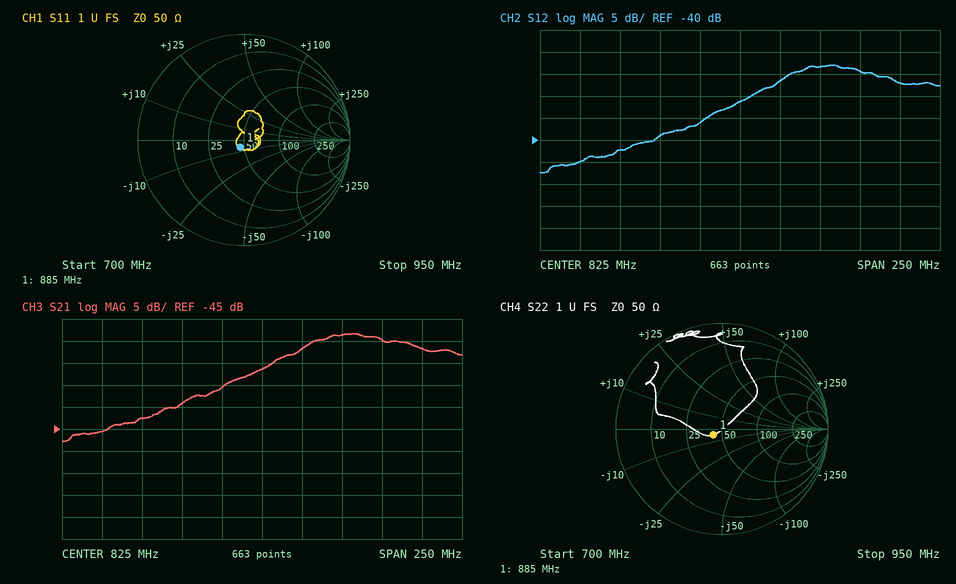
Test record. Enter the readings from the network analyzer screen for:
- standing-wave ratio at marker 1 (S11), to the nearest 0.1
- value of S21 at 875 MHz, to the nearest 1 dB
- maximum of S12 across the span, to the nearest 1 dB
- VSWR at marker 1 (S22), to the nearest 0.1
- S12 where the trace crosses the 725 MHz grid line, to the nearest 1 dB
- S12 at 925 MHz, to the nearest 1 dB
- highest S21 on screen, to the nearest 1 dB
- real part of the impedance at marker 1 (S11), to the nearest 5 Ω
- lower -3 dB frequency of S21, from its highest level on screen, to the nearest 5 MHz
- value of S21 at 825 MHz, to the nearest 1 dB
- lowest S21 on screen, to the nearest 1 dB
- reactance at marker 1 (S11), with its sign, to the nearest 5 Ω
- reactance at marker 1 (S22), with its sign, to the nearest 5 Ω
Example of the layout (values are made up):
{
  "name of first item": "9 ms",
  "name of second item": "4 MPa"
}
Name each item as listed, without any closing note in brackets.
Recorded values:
{
  "standing-wave ratio at marker 1 (S11), to the nearest 0.1": "1.2",
  "value of S21 at 875 MHz, to the nearest 1 dB": "-24 dB",
  "maximum of S12 across the span, to the nearest 1 dB": "-23 dB",
  "VSWR at marker 1 (S22), to the nearest 0.1": "1.2",
  "S12 where the trace crosses the 725 MHz grid line, to the nearest 1 dB": "-45 dB",
  "S12 at 925 MHz, to the nearest 1 dB": "-27 dB",
  "highest S21 on screen, to the nearest 1 dB": "-23 dB",
  "real part of the impedance at marker 1 (S11), to the nearest 5 Ω": "45 Ω",
  "lower -3 dB frequency of S21, from its highest level on screen, to the nearest 5 MHz": "850 MHz",
  "value of S21 at 825 MHz, to the nearest 1 dB": "-31 dB",
  "lowest S21 on screen, to the nearest 1 dB": "-48 dB",
  "reactance at marker 1 (S11), with its sign, to the nearest 5 Ω": "-5 Ω",
  "reactance at marker 1 (S22), with its sign, to the nearest 5 Ω": "-5 Ω"
}
